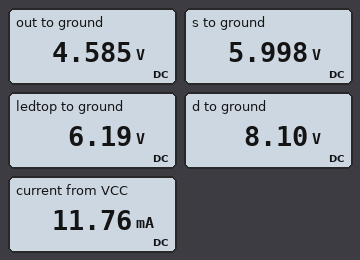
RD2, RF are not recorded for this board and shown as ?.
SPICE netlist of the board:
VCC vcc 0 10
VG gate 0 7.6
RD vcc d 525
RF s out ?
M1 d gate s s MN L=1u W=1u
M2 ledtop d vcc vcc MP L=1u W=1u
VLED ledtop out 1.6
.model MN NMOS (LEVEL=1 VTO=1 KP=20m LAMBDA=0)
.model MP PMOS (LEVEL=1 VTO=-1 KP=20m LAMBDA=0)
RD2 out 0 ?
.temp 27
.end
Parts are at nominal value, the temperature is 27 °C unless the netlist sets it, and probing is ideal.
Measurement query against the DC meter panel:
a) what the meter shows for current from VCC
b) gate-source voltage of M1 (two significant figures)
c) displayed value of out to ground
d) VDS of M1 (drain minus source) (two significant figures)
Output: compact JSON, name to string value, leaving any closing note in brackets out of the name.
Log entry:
{"what the meter shows for current from VCC": "11.76 mA", "gate-source voltage of M1": "1.6 V", "displayed value of out to ground": "4.585 V", "VDS of M1 (drain minus source)": "2.1 V"}
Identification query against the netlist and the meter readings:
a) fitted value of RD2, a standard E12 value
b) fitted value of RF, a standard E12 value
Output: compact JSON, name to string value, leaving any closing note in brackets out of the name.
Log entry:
{"fitted value of RD2, a standard E12 value": "390 Ω", "fitted value of RF, a standard E12 value": "390 Ω"}
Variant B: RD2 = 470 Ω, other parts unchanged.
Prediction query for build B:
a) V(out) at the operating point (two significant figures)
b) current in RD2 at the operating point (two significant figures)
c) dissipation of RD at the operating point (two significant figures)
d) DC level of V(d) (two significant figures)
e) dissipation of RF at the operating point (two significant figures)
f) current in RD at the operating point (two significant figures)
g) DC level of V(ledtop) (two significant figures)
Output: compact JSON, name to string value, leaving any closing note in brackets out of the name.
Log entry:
{"V(out) at the operating point": "4.7 V", "current in RD2 at the operating point": "9.9 mA", "dissipation of RD at the operating point": "6.2 mW", "DC level of V(d)": "8.2 V", "dissipation of RF at the operating point": "4.6 mW", "current in RD at the operating point": "3.4 mA", "DC level of V(ledtop)": "6.3 V"}
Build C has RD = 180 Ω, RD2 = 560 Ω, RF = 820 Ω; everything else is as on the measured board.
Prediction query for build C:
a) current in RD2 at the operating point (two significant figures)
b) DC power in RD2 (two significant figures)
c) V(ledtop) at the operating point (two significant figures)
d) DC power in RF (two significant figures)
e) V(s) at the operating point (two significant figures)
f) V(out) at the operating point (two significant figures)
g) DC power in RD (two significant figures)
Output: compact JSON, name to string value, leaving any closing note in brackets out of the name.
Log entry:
{"current in RD2 at the operating point": "4.3 mA", "DC power in RD2": "10 mW", "V(ledtop) at the operating point": "4.0 V", "DC power in RF": "15 mW", "V(s) at the operating point": "5.9 V", "V(out) at the operating point": "2.4 V", "DC power in RD": "3.3 mW"}
